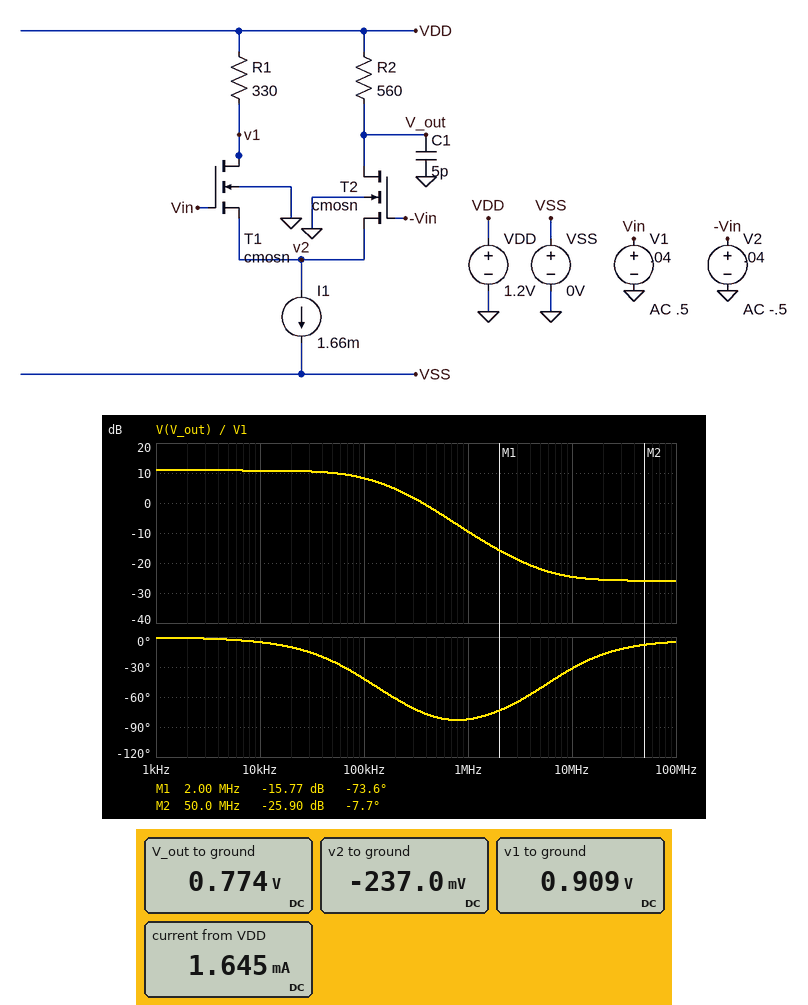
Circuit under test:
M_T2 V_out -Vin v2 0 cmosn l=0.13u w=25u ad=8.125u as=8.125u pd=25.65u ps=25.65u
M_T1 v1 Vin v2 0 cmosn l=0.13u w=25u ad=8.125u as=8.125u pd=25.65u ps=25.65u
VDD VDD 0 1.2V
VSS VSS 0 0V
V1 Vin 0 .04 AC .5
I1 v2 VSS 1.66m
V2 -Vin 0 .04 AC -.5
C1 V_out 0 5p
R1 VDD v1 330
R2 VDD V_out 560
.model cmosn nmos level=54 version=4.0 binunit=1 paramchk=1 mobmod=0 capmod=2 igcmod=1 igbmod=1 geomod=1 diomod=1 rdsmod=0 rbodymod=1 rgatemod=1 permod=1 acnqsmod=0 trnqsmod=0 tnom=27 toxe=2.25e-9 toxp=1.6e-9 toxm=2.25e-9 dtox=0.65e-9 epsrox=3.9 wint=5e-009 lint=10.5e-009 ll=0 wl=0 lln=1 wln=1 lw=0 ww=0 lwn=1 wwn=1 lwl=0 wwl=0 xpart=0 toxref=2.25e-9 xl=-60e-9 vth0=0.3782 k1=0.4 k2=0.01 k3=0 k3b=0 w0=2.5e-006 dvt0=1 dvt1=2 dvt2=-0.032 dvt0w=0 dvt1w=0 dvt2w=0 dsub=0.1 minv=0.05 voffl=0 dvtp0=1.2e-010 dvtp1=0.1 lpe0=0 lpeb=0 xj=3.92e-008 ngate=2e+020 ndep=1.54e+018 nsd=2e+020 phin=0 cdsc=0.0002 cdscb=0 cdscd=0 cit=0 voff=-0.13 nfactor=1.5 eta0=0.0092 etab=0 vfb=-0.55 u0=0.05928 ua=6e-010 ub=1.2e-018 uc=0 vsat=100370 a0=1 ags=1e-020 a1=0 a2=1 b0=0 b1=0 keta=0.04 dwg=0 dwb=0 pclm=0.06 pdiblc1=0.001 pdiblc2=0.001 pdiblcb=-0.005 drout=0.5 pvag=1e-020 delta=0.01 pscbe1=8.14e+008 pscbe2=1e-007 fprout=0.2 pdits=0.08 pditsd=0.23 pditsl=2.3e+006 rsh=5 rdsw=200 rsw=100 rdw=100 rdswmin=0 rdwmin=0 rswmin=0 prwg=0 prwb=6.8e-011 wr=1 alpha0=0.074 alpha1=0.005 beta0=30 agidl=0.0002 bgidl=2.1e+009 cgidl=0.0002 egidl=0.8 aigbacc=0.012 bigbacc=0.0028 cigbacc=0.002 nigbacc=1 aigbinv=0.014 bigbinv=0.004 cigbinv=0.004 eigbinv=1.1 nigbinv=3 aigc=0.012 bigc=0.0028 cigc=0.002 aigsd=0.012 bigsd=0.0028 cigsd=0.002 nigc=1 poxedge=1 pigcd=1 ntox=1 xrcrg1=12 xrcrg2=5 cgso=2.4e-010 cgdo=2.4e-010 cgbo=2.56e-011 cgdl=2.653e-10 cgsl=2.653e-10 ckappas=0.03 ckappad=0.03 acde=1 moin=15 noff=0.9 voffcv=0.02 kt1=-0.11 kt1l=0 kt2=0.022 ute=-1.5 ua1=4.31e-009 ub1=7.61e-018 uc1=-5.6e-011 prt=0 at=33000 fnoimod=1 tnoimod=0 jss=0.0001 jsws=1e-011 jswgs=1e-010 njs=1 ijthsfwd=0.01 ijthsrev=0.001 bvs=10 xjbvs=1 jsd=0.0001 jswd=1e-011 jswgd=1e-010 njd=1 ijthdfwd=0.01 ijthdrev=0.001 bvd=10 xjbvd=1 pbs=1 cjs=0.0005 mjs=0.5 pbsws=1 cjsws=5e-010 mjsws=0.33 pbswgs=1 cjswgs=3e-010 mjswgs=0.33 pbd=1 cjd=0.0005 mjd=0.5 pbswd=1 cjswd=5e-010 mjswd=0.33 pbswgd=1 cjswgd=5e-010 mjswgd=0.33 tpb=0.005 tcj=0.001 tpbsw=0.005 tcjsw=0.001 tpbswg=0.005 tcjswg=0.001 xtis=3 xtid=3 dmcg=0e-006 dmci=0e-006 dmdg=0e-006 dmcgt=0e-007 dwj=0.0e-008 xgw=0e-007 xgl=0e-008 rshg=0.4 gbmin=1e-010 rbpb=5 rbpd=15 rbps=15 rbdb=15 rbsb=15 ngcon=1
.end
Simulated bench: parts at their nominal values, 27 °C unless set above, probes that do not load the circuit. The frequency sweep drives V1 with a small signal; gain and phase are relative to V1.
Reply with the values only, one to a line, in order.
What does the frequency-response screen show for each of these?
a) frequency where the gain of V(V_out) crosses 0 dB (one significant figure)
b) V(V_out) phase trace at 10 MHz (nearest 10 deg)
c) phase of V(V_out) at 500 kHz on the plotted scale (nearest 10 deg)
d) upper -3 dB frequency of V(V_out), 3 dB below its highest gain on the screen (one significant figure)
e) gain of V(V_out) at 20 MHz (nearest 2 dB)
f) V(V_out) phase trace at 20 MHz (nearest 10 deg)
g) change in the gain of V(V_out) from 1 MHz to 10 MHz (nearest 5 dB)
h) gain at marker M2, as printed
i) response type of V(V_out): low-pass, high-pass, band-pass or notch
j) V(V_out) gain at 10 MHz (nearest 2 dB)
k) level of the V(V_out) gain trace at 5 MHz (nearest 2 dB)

400 kHz
-30 deg
-80 deg
100 kHz
-26 dB
-20 deg
-15 dB
-25.90 dB
low-pass
-24 dB
-22 dB
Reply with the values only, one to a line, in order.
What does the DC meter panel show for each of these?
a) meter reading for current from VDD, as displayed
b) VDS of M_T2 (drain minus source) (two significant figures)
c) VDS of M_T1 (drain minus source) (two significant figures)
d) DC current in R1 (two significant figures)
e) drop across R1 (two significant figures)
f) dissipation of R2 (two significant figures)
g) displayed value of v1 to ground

1.645 mA
1.0 V
1.1 V
880 µA
290 mV
320 µW
0.909 V
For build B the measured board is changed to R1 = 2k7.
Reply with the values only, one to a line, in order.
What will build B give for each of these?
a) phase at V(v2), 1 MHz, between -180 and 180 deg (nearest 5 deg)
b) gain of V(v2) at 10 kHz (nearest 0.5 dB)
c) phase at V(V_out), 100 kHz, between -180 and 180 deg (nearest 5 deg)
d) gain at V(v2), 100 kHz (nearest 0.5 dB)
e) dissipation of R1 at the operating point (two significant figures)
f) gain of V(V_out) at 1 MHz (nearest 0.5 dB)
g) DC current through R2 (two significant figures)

-60 deg
-19.0 dB
-35 deg
-24.5 dB
650 µW
-9.0 dB
1.1 mA
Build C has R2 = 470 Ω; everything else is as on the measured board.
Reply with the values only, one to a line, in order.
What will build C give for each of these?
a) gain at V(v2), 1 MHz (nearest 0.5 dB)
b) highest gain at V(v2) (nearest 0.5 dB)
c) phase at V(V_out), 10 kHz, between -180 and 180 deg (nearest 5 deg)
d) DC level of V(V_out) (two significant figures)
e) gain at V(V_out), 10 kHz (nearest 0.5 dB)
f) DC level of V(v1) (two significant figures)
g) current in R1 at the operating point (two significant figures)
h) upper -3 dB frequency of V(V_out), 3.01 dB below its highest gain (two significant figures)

-21.0 dB
-13.0 dB
-5 deg
830 mV
9.5 dB
920 mV
860 µA
130 kHz
